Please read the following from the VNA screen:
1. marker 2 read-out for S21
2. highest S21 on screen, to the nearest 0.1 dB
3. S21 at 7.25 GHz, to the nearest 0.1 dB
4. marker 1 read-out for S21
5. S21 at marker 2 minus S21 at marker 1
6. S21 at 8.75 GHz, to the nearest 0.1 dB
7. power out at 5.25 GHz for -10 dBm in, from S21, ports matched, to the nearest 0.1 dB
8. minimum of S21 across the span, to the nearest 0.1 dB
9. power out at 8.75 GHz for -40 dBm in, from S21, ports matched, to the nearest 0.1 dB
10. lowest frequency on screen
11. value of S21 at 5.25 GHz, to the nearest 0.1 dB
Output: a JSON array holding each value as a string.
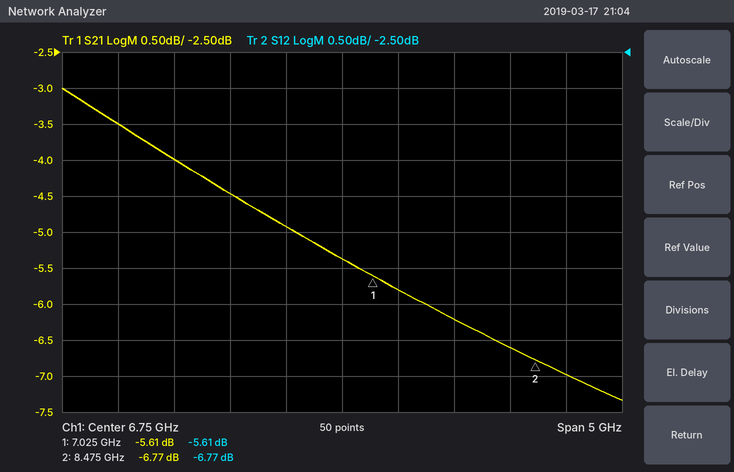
["-6.77 dB", "-3.0 dB", "-5.8 dB", "-5.61 dB", "-1.16 dB", "-7.0 dB", "-14.0 dBm", "-7.3 dB", "-47.0 dBm", "4.25 GHz", "-4.0 dB"]
